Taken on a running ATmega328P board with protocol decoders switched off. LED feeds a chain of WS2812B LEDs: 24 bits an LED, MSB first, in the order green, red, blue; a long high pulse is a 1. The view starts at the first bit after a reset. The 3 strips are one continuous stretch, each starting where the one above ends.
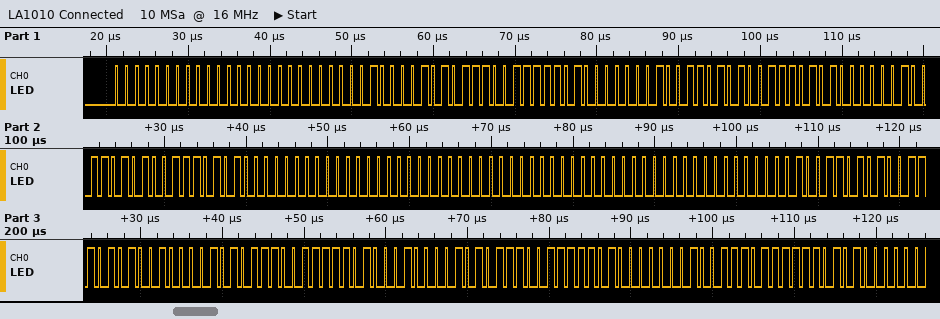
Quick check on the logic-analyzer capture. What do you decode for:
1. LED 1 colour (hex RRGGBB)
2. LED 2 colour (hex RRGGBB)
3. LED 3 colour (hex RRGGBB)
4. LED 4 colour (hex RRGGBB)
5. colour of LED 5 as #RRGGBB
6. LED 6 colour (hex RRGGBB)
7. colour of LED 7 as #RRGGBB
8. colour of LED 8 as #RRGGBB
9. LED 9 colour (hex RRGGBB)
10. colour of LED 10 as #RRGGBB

#000000
#B942F4
#D404EA
#D404EA
#000000
#000000
#D404EA
#B942F4
#B942F4
#EF04D4
